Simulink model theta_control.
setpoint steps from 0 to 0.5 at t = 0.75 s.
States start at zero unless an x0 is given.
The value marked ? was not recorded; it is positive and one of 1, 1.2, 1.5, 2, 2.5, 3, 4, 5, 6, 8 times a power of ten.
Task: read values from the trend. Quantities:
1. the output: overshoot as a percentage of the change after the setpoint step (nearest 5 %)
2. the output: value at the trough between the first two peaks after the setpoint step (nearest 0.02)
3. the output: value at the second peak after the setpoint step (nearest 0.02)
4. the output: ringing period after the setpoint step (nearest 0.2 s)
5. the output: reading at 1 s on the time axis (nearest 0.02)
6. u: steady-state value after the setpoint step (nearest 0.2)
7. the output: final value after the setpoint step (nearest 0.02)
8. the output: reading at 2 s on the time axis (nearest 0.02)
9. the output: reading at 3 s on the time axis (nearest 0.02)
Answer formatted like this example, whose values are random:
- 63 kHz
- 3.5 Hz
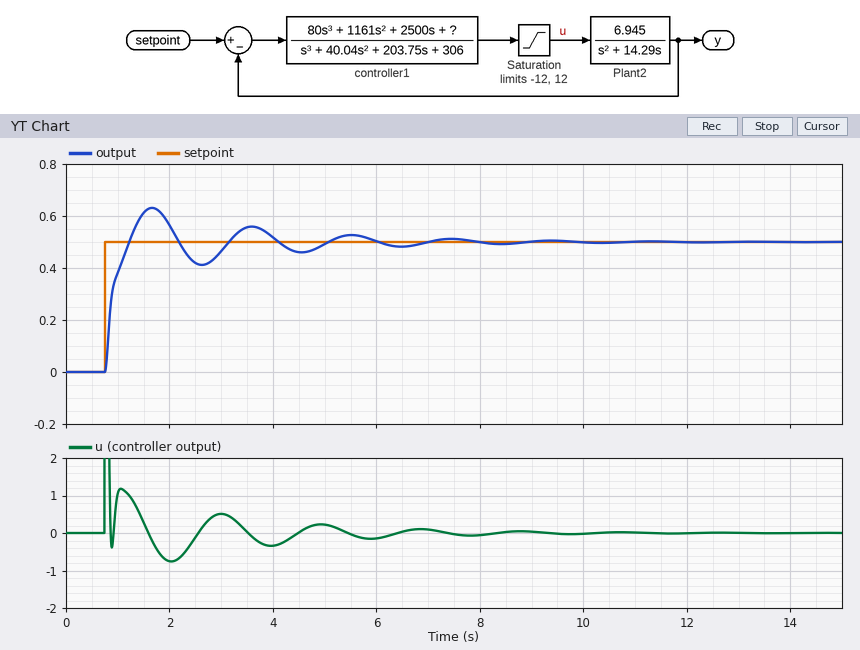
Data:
- 25 %
- 0.42
- 0.56
- 2.0 s
- 0.38
- 0.0
- 0.50
- 0.56
- 0.46
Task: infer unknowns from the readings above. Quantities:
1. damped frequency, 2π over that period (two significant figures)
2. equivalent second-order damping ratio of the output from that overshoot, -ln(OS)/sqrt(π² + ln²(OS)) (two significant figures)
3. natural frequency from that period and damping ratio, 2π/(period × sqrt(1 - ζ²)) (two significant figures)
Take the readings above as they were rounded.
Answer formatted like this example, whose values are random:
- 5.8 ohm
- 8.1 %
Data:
- 3.1 rad/s
- 0.40
- 3.4 rad/s
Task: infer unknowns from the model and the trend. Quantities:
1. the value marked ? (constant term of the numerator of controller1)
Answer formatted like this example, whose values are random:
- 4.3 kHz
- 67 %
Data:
- 15000
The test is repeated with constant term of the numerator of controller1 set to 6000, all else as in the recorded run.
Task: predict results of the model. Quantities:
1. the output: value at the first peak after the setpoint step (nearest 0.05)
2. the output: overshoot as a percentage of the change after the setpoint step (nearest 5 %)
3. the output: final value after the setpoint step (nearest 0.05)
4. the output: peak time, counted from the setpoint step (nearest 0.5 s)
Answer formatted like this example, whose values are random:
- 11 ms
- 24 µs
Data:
- 0.55
- 10 %
- 0.50
- 1.5 s
